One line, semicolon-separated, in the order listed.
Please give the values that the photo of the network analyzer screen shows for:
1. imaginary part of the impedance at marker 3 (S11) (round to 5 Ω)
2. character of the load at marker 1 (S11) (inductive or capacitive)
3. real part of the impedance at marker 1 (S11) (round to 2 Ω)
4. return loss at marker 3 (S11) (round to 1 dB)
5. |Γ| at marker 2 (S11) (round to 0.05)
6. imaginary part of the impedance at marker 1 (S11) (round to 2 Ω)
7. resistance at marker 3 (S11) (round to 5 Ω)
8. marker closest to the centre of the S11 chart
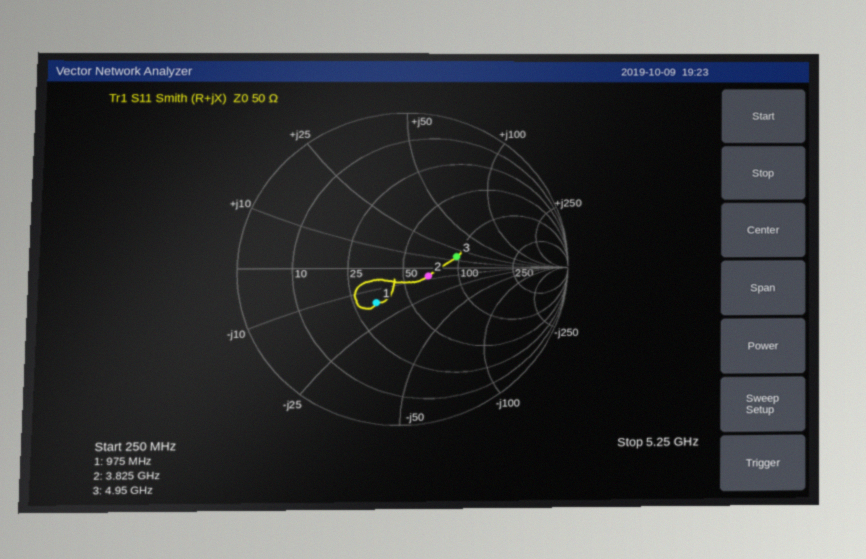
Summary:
+15 Ω; capacitive; 34 Ω; 10 dB; 0.15; -16 Ω; 95 Ω; marker 2
